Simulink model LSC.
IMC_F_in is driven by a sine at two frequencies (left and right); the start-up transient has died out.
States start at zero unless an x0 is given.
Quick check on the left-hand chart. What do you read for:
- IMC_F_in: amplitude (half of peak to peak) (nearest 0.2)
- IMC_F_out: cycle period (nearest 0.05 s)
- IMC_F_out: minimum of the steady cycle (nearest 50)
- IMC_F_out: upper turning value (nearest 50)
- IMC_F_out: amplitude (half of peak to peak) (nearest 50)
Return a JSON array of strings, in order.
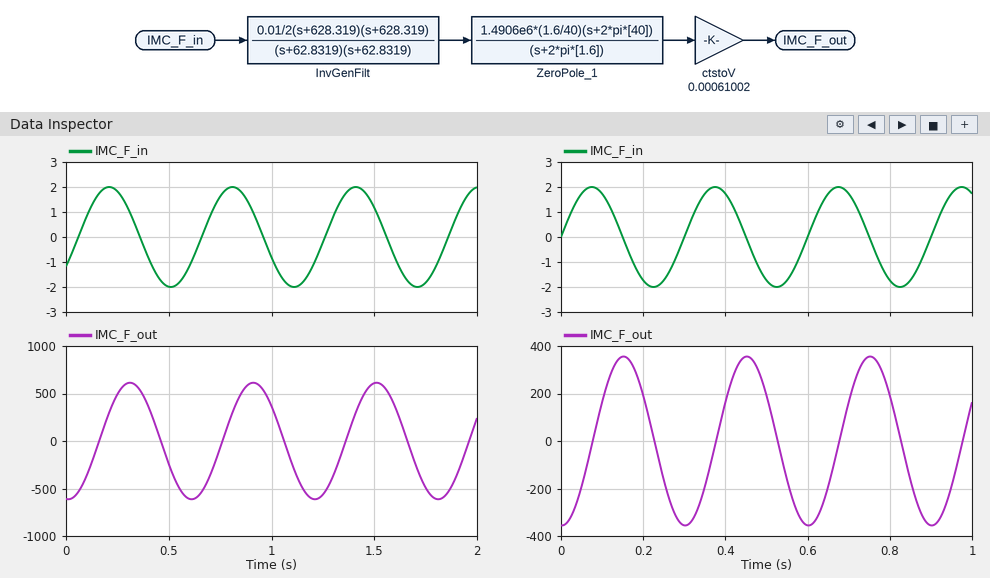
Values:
["2.0", "0.60 s", "-600", "600", "600"]
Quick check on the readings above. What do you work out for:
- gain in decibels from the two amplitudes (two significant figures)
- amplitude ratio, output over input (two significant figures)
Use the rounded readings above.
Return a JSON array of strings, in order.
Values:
["50 dB", "300"]
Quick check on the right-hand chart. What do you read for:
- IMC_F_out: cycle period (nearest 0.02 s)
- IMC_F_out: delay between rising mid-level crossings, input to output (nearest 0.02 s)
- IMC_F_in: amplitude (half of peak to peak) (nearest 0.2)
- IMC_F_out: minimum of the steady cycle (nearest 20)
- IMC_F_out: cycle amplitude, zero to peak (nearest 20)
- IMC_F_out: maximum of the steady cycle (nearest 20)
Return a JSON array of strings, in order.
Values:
["0.30 s", "0.08 s", "2.0", "-360", "360", "360"]
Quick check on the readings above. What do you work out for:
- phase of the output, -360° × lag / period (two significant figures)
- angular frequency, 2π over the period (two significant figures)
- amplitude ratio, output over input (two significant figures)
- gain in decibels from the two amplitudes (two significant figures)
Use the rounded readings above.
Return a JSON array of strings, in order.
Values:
["-96°", "21 rad/s", "180", "45 dB"]
